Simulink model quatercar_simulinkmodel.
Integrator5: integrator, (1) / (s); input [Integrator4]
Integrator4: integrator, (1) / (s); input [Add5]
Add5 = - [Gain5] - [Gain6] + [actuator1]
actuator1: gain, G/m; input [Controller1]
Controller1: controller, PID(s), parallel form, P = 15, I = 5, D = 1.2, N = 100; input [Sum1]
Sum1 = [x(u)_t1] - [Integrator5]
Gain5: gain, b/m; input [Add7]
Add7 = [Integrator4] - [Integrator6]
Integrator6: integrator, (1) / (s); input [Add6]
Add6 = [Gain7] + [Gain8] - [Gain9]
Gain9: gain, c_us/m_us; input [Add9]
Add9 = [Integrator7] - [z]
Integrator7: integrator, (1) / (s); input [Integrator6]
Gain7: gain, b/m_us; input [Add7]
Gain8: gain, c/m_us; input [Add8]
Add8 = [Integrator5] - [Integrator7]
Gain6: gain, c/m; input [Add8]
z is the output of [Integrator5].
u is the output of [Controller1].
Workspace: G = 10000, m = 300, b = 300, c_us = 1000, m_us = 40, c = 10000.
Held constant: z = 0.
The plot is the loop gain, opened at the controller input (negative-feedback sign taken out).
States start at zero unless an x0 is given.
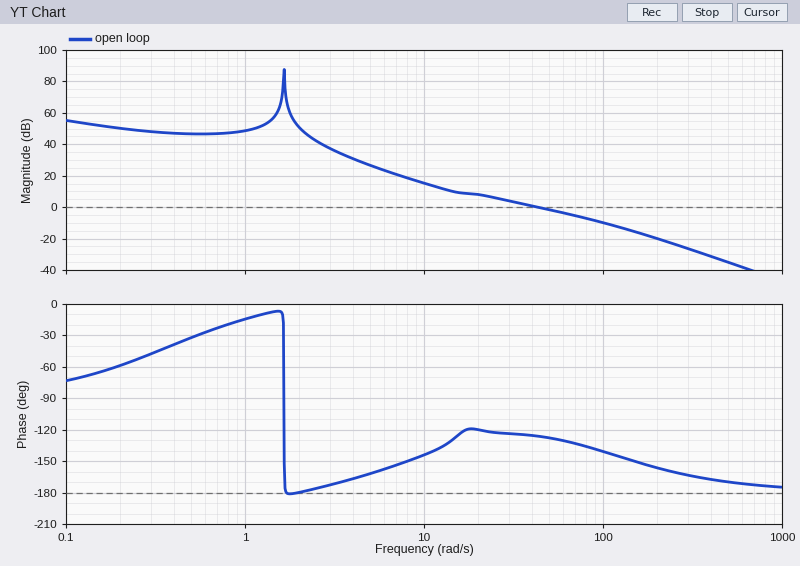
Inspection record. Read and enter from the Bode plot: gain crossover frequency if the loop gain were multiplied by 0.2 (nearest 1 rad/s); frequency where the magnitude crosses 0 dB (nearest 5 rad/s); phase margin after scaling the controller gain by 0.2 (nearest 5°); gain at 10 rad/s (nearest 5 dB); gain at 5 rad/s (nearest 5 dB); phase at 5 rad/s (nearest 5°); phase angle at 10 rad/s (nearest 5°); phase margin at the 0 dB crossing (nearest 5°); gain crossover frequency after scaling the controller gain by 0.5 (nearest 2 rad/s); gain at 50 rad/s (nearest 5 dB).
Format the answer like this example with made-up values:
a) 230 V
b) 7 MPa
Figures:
a) 11 rad/s
b) 45 rad/s
c) 40°
d) 15 dB
e) 25 dB
f) -160°
g) -145°
h) 55°
i) 24 rad/s
j) 0 dB
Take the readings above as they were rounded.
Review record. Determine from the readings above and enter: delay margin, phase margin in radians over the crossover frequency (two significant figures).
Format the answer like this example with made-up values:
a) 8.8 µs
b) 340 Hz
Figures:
a) 0.021 s
